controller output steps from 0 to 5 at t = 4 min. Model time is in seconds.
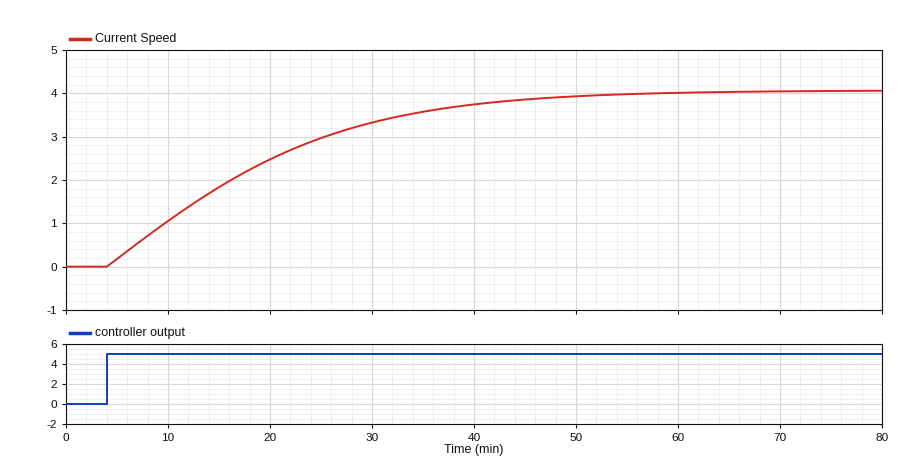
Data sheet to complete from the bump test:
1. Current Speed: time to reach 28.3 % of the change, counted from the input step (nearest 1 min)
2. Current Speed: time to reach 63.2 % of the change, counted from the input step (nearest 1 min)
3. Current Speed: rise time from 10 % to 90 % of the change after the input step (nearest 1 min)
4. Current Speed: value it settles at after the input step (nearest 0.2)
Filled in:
7 min
17 min
31 min
4.0
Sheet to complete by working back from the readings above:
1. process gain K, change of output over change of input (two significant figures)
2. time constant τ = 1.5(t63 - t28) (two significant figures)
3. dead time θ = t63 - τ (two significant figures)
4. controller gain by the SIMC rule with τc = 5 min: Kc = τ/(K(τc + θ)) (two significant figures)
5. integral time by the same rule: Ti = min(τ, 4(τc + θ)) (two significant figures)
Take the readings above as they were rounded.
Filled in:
0.80
15 min
2.0 min
2.7
15 min
